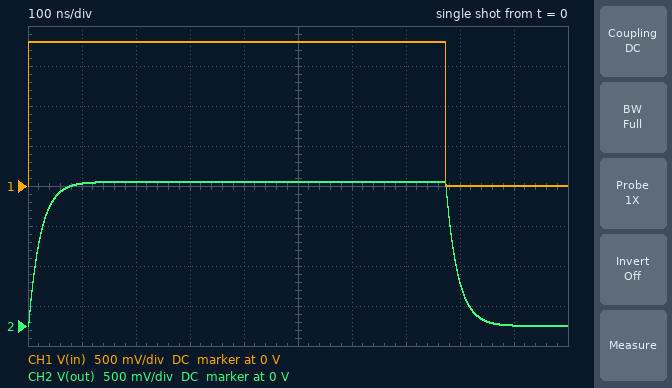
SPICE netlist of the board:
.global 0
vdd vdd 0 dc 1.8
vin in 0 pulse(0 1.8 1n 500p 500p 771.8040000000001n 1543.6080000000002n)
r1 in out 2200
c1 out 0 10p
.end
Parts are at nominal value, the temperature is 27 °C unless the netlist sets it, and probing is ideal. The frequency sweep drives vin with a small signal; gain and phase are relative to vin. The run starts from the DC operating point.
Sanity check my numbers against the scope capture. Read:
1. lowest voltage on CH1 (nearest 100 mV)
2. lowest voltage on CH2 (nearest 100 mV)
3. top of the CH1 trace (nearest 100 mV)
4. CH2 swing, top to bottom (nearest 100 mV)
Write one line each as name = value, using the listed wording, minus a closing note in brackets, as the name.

lowest voltage on CH1 = 0 V
lowest voltage on CH2 = 0 V
top of the CH1 trace = 1.8 V
CH2 swing, top to bottom = 1.8 V
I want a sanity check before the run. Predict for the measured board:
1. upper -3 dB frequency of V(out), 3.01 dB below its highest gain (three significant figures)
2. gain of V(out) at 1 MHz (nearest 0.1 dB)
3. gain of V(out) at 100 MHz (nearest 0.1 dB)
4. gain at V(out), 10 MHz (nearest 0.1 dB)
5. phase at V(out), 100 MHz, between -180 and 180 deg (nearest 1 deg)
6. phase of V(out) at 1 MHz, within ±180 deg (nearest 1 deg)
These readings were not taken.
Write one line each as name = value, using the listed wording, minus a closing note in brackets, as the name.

upper -3 dB frequency of V(out), 3.01 dB below its highest gain = 7.23 MHz
gain of V(out) at 1 MHz = -0.1 dB
gain of V(out) at 100 MHz = -22.8 dB
gain at V(out), 10 MHz = -4.6 dB
phase at V(out), 100 MHz, between -180 and 180 deg = -86 deg
phase of V(out) at 1 MHz, within ±180 deg = -8 deg
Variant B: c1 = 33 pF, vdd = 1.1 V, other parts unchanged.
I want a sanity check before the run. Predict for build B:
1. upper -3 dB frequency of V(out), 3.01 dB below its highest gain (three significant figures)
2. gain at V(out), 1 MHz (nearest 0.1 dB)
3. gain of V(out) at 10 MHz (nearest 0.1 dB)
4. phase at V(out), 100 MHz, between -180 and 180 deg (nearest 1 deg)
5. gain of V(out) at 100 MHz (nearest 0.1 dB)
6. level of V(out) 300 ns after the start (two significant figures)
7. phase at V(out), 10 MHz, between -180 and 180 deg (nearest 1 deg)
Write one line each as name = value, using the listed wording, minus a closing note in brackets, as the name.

upper -3 dB frequency of V(out), 3.01 dB below its highest gain = 2.19 MHz
gain at V(out), 1 MHz = -0.8 dB
gain of V(out) at 10 MHz = -13.4 dB
phase at V(out), 100 MHz, between -180 and 180 deg = -89 deg
gain of V(out) at 100 MHz = -33.2 dB
level of V(out) 300 ns after the start = 1.8 V
phase at V(out), 10 MHz, between -180 and 180 deg = -78 deg
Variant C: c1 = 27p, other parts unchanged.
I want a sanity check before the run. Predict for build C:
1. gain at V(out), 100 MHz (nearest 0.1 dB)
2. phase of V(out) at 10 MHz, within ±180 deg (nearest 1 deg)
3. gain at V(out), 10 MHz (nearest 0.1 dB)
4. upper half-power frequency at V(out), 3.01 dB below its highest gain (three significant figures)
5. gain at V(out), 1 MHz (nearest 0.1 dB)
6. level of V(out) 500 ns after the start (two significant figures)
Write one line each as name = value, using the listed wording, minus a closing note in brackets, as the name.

gain at V(out), 100 MHz = -31.4 dB
phase of V(out) at 10 MHz, within ±180 deg = -75 deg
gain at V(out), 10 MHz = -11.7 dB
upper half-power frequency at V(out), 3.01 dB below its highest gain = 2.68 MHz
gain at V(out), 1 MHz = -0.6 dB
level of V(out) 500 ns after the start = 1.8 V
